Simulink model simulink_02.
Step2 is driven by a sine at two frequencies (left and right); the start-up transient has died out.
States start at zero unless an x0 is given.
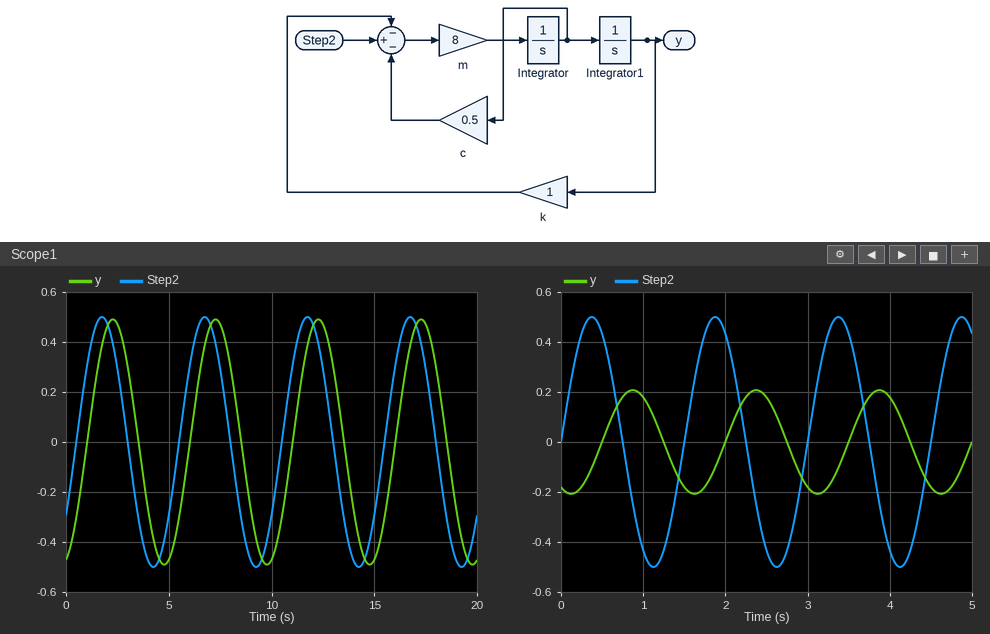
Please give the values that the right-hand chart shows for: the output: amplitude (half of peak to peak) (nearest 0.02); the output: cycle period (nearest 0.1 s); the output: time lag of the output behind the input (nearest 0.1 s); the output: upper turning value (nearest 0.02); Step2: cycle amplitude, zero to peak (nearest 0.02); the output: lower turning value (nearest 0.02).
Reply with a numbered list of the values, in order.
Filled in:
1. 0.20
2. 1.5 s
3. 0.5 s
4. 0.20
5. 0.50
6. -0.20
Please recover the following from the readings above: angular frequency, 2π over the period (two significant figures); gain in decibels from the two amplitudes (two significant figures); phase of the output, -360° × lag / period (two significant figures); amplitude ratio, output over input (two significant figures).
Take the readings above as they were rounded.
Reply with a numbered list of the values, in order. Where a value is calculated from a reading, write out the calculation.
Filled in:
1. 2π / 1.5 = 4.2 rad/s
2. 20 log10(0.2 / 0.5) = -8.0 dB
3. -360 × 0.5 / 1.5 = -120°
4. 0.2 / 0.5 = 0.40
